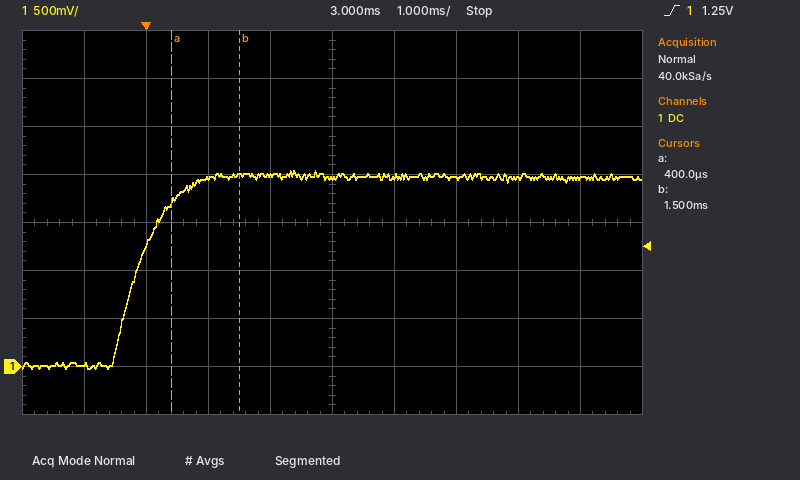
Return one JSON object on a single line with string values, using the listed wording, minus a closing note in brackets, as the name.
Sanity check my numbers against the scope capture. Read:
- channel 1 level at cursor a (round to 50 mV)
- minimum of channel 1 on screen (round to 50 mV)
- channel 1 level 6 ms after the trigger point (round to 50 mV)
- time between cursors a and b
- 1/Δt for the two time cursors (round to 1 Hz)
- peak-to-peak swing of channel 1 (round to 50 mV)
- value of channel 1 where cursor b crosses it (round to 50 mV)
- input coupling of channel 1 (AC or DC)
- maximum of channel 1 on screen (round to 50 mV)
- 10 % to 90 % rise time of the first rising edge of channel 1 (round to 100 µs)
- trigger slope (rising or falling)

{"channel 1 level at cursor a": "1.70 V", "minimum of channel 1 on screen": "0 mV", "channel 1 level 6 ms after the trigger point": "1.95 V", "time between cursors a and b": "1.1 ms", "1/Δt for the two time cursors": "909 Hz", "peak-to-peak swing of channel 1": "2.05 V", "value of channel 1 where cursor b crosses it": "2.00 V", "input coupling of channel 1": "DC", "maximum of channel 1 on screen": "2.05 V", "10 % to 90 % rise time of the first rising edge of channel 1": "1.0 ms", "trigger slope": "rising"}
